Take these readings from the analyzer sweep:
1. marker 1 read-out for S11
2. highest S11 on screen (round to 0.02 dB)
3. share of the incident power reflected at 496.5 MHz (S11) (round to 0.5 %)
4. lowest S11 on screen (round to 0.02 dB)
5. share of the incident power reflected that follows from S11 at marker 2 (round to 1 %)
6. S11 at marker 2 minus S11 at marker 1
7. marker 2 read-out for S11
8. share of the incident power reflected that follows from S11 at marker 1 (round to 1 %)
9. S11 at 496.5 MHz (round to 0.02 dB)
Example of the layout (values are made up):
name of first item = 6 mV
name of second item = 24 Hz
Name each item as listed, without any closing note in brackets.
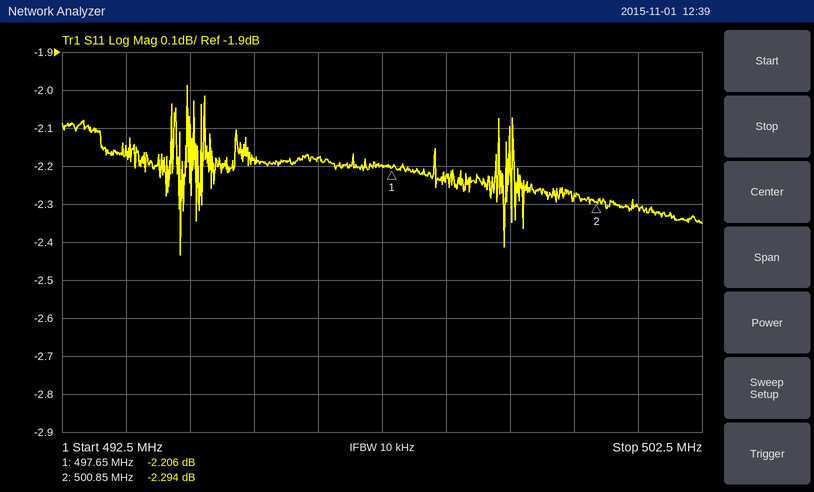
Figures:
marker 1 read-out for S11 = -2.206 dB
highest S11 on screen = -1.98 dB
share of the incident power reflected at 496.5 MHz (S11) = 60.5 %
lowest S11 on screen = -2.44 dB
share of the incident power reflected that follows from S11 at marker 2 = 59 %
S11 at marker 2 minus S11 at marker 1 = -0.088 dB
marker 2 read-out for S11 = -2.294 dB
share of the incident power reflected that follows from S11 at marker 1 = 60 %
S11 at 496.5 MHz = -2.18 dB
